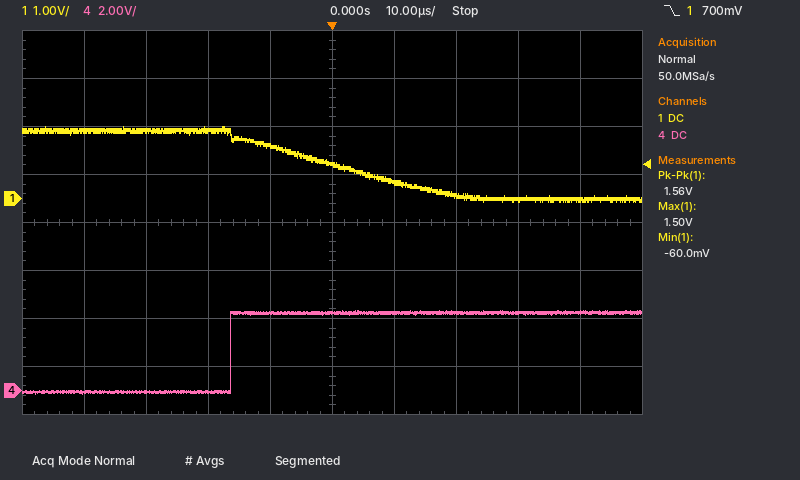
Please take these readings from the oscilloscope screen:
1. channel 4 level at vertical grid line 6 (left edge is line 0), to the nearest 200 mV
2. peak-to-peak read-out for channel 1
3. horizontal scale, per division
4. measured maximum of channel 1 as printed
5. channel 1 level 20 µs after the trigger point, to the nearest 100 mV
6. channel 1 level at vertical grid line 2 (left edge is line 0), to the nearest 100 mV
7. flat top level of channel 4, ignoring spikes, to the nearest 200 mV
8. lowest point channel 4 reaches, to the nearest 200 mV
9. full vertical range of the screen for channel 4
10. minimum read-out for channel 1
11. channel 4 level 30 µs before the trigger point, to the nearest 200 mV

3.2 V
1.56 V
10 µs
1.50 V
100 mV
1.4 V
3.2 V
-200 mV
16 V
-60.0 mV
0.0 V
